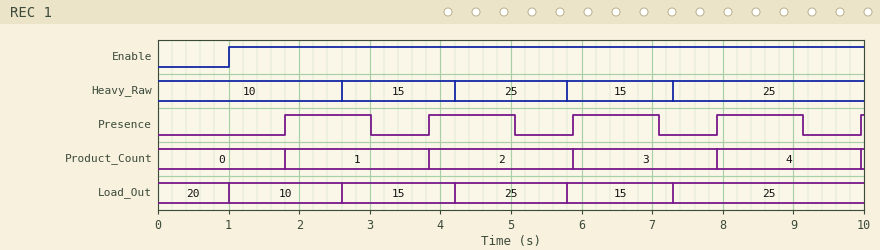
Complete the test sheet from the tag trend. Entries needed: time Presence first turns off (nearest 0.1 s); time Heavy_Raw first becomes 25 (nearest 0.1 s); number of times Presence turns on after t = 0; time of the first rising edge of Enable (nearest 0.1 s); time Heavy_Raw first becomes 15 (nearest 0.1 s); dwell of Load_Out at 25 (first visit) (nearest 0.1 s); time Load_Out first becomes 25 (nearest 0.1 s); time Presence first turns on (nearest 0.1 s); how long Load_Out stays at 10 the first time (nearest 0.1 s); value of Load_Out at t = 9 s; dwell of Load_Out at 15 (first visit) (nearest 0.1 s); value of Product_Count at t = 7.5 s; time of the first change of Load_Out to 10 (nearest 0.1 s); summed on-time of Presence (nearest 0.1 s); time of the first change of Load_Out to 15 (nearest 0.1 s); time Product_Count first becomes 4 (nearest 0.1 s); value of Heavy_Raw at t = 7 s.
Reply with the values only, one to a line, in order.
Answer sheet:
3.0 s
4.2 s
5
1.0 s
2.6 s
1.6 s
4.2 s
1.8 s
1.6 s
25
1.6 s
3
1.0 s
4.9 s
2.6 s
7.9 s
15
